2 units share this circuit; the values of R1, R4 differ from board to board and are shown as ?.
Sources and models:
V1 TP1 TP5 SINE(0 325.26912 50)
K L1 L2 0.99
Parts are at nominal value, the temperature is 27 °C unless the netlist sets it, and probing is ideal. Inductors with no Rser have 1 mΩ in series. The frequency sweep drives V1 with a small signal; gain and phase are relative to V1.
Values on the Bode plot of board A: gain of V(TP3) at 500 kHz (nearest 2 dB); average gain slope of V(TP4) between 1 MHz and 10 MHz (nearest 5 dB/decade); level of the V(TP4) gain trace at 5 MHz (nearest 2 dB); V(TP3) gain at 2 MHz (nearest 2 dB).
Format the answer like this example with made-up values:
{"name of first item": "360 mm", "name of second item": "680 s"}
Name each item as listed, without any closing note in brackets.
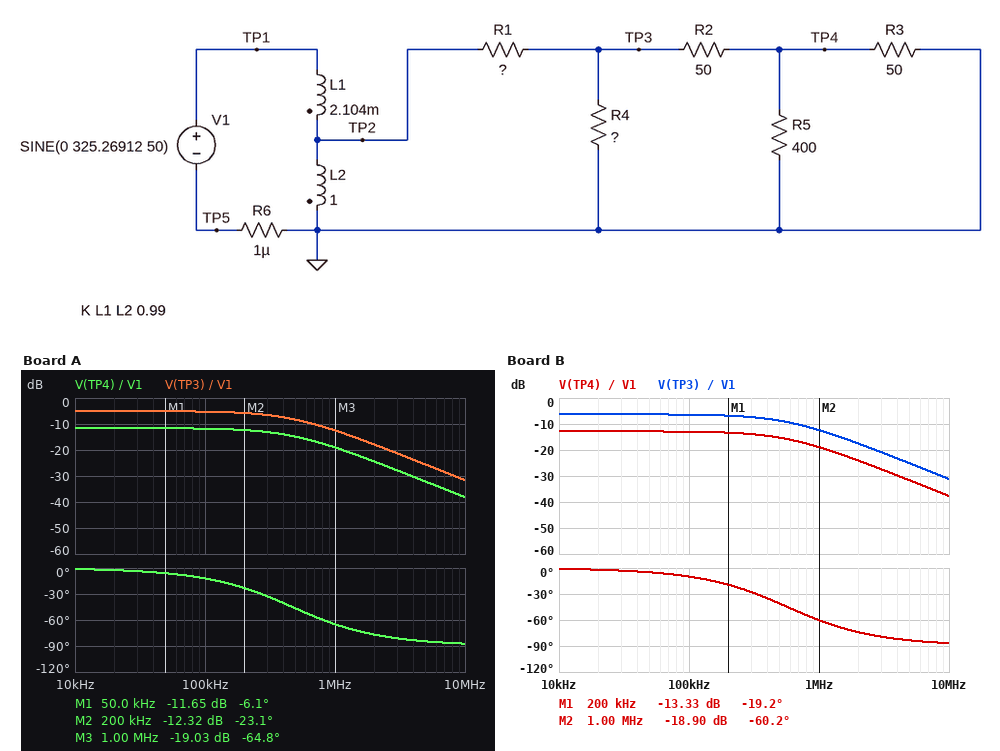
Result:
{"gain of V(TP3) at 500 kHz": "-8 dB", "average gain slope of V(TP4) between 1 MHz and 10 MHz": "-20 dB/decade", "level of the V(TP4) gain trace at 5 MHz": "-32 dB", "V(TP3) gain at 2 MHz": "-18 dB"}
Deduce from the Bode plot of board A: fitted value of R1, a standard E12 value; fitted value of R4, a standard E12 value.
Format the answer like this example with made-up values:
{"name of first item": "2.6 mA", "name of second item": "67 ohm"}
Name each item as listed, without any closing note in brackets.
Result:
{"fitted value of R1, a standard E12 value": "47 Ω", "fitted value of R4, a standard E12 value": "220 Ω"}
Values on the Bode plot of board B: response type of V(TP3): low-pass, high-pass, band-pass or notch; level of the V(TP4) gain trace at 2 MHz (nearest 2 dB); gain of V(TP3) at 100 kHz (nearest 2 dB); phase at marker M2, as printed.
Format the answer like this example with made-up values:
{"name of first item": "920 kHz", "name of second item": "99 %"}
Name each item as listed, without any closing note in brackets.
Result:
{"response type of V(TP3): low-pass, high-pass, band-pass or notch": "low-pass", "level of the V(TP4) gain trace at 2 MHz": "-24 dB", "gain of V(TP3) at 100 kHz": "-6 dB", "phase at marker M2, as printed": "-60.2 deg"}
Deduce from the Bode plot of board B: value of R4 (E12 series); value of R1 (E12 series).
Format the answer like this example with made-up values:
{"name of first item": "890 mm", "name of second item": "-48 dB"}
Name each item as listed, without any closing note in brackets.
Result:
{"value of R4": "270 Ω", "value of R1": "68 Ω"}
